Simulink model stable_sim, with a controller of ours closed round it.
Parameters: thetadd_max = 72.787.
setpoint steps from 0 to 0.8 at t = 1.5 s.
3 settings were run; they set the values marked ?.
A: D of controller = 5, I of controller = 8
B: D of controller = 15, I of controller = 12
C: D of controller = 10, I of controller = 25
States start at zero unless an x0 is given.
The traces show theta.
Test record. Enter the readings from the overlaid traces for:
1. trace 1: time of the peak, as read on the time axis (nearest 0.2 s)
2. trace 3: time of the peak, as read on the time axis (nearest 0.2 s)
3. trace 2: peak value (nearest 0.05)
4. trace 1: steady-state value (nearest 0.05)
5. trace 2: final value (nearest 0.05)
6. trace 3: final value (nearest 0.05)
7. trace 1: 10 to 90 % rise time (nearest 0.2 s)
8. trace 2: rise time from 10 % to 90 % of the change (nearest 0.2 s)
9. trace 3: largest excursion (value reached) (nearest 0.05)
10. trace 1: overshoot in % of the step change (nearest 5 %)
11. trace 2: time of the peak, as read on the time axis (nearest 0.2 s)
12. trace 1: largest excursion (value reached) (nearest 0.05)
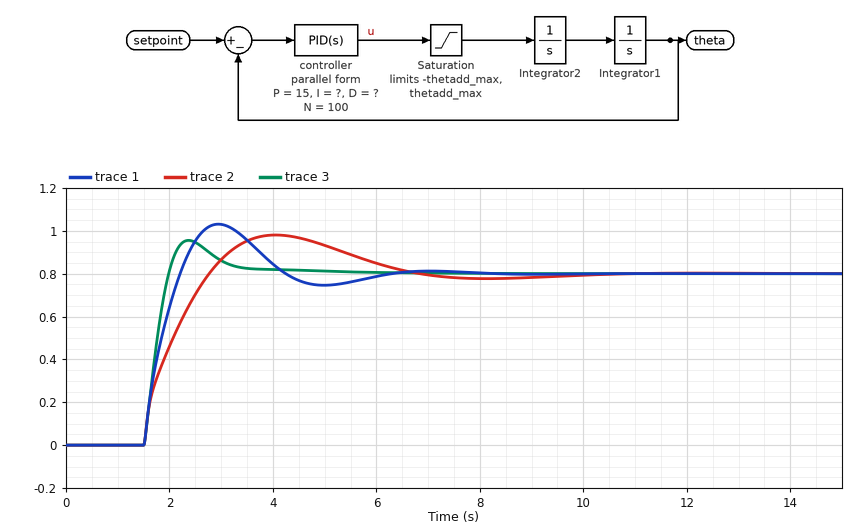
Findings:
3.0 s
2.4 s
1.00
0.80
0.80
0.80
0.6 s
1.0 s
0.95
30 %
4.0 s
1.05
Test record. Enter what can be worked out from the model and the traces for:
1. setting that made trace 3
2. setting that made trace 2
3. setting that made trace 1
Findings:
A
B
C
